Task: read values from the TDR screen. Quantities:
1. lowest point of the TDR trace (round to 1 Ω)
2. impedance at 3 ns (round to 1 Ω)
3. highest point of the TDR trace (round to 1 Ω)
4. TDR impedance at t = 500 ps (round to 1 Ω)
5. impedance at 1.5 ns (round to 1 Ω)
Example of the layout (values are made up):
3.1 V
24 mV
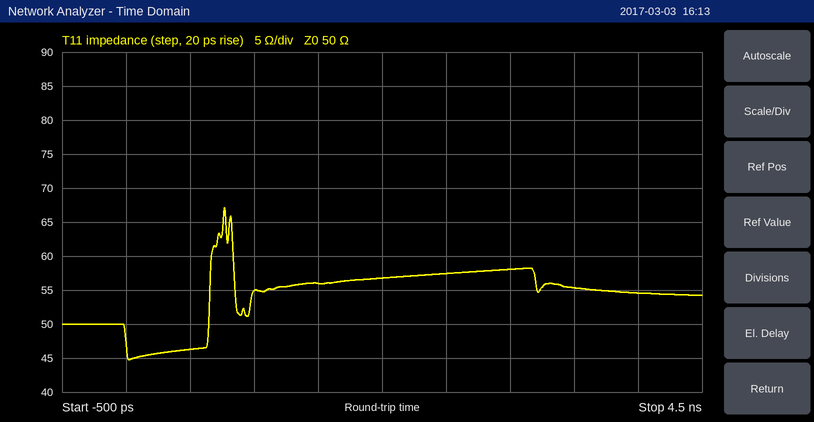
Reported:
45 Ω
58 Ω
67 Ω
46 Ω
56 Ω
